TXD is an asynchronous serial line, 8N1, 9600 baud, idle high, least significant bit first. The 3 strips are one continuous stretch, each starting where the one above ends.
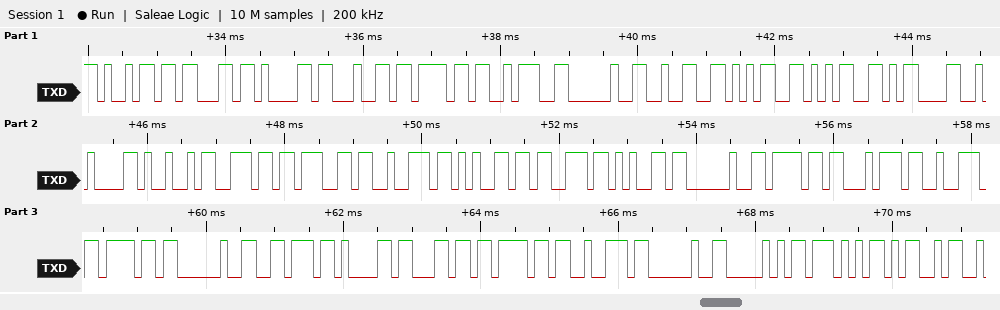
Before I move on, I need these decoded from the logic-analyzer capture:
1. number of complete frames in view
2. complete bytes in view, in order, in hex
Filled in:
34
69 63 61 64 6F 3A 20 32 35 35 0D 0A 49 6E 67 72 65 73 65 20 6F 74 72 6F 20 76 61 6C 6F 72 20 50 57 4D
